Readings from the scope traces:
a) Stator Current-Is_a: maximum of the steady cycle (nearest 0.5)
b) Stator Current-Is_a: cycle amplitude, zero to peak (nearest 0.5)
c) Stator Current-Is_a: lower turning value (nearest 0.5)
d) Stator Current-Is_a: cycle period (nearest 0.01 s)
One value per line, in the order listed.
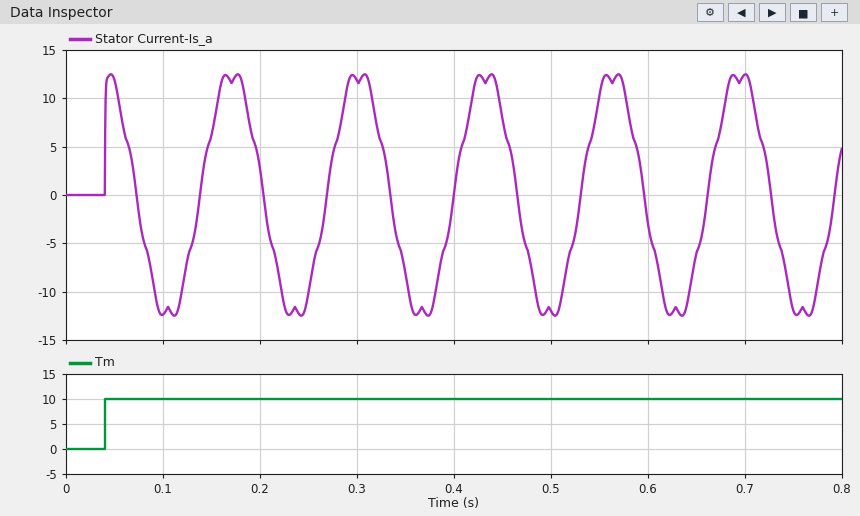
12.5
12.5
-12.5
0.13 s
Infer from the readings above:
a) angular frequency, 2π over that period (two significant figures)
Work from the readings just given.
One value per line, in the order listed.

48 rad/s
